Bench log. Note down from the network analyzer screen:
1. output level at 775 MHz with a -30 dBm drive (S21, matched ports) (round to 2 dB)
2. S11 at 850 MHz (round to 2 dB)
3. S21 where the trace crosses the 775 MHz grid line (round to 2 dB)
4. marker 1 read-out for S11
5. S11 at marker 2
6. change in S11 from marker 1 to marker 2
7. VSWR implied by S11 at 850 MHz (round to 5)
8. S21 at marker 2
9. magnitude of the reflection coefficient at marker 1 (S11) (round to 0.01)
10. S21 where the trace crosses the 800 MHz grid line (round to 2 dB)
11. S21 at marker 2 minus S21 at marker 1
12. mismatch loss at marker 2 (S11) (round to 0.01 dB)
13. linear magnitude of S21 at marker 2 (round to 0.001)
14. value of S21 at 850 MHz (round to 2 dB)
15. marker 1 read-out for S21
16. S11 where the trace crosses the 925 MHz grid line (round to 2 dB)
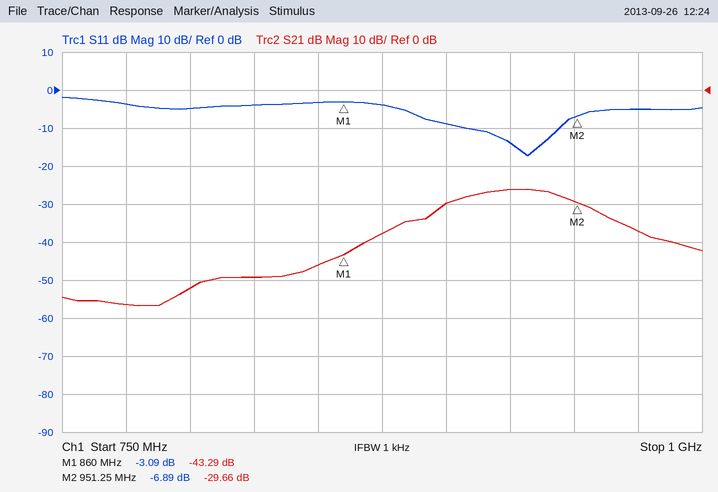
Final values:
-86 dBm
-4 dB
-56 dB
-3.09 dB
-6.89 dB
-3.80 dB
5
-29.66 dB
0.70
-52 dB
13.63 dB
0.99 dB
0.033
-46 dB
-43.29 dB
-14 dB
